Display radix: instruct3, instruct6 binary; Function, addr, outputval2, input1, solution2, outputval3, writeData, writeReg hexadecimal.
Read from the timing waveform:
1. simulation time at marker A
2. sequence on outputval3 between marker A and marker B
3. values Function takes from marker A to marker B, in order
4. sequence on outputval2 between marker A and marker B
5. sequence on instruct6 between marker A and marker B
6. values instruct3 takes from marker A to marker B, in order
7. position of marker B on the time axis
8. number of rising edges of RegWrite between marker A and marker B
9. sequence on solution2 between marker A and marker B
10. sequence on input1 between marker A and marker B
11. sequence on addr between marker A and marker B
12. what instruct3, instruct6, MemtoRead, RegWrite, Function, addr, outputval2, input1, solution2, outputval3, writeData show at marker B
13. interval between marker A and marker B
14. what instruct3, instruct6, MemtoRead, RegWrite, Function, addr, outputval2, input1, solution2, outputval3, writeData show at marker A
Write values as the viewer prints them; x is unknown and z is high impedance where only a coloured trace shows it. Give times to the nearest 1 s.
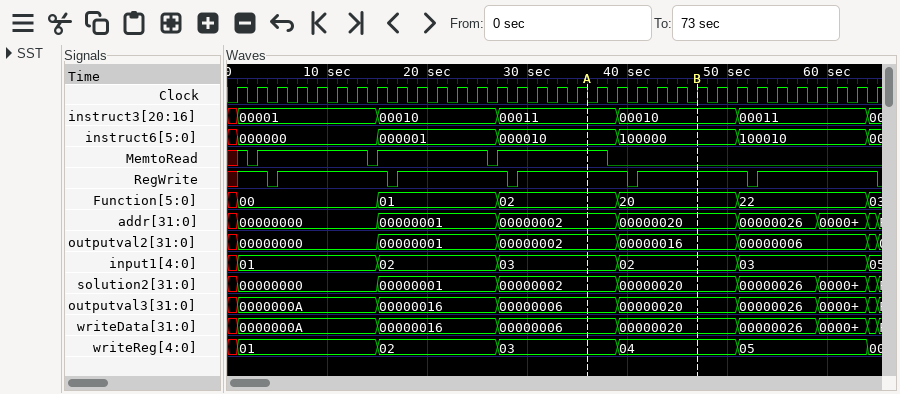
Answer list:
36 s
00000006, 00000020
02, 20
00000002, 00000016
000010, 100000
00011, 00010
47 s
1
00000002, 00000020
03, 02
00000002, 00000020
instruct3=00010, instruct6=100000, MemtoRead=0, RegWrite=1, Function=20, addr=00000020, outputval2=00000016, input1=02, solution2=00000020, outputval3=00000020, writeData=00000020
11 s
instruct3=00011, instruct6=000010, MemtoRead=1, RegWrite=1, Function=02, addr=00000002, outputval2=00000002, input1=03, solution2=00000002, outputval3=00000006, writeData=00000006
